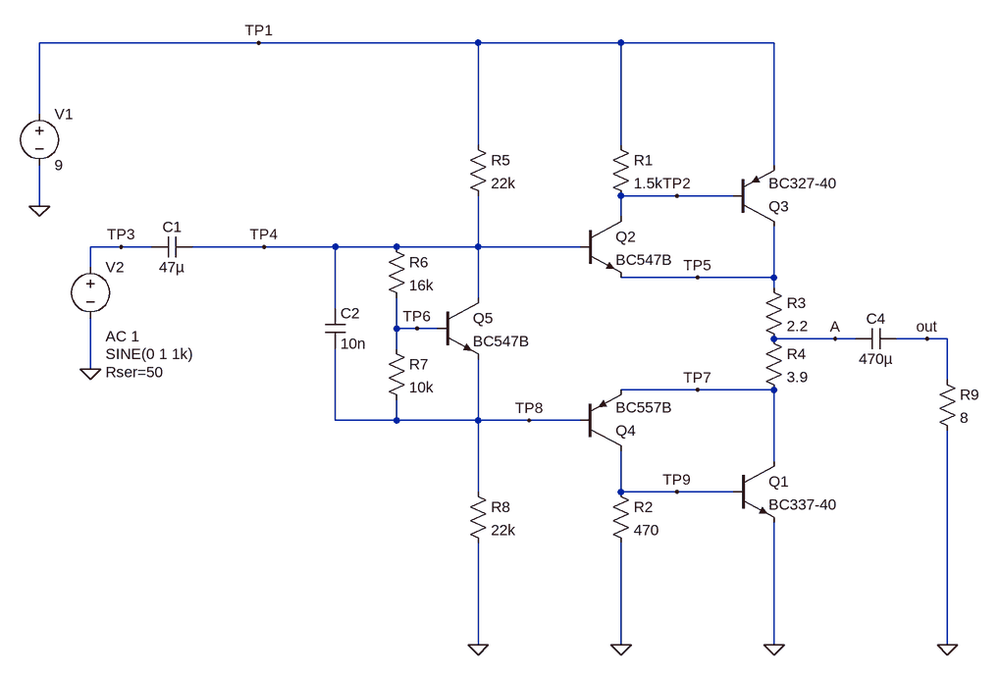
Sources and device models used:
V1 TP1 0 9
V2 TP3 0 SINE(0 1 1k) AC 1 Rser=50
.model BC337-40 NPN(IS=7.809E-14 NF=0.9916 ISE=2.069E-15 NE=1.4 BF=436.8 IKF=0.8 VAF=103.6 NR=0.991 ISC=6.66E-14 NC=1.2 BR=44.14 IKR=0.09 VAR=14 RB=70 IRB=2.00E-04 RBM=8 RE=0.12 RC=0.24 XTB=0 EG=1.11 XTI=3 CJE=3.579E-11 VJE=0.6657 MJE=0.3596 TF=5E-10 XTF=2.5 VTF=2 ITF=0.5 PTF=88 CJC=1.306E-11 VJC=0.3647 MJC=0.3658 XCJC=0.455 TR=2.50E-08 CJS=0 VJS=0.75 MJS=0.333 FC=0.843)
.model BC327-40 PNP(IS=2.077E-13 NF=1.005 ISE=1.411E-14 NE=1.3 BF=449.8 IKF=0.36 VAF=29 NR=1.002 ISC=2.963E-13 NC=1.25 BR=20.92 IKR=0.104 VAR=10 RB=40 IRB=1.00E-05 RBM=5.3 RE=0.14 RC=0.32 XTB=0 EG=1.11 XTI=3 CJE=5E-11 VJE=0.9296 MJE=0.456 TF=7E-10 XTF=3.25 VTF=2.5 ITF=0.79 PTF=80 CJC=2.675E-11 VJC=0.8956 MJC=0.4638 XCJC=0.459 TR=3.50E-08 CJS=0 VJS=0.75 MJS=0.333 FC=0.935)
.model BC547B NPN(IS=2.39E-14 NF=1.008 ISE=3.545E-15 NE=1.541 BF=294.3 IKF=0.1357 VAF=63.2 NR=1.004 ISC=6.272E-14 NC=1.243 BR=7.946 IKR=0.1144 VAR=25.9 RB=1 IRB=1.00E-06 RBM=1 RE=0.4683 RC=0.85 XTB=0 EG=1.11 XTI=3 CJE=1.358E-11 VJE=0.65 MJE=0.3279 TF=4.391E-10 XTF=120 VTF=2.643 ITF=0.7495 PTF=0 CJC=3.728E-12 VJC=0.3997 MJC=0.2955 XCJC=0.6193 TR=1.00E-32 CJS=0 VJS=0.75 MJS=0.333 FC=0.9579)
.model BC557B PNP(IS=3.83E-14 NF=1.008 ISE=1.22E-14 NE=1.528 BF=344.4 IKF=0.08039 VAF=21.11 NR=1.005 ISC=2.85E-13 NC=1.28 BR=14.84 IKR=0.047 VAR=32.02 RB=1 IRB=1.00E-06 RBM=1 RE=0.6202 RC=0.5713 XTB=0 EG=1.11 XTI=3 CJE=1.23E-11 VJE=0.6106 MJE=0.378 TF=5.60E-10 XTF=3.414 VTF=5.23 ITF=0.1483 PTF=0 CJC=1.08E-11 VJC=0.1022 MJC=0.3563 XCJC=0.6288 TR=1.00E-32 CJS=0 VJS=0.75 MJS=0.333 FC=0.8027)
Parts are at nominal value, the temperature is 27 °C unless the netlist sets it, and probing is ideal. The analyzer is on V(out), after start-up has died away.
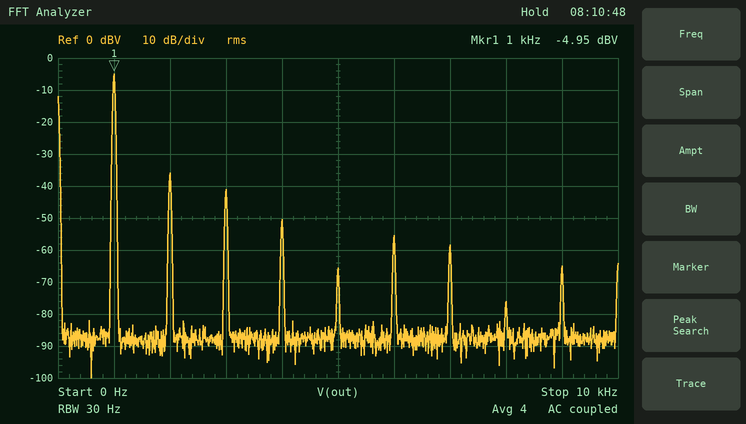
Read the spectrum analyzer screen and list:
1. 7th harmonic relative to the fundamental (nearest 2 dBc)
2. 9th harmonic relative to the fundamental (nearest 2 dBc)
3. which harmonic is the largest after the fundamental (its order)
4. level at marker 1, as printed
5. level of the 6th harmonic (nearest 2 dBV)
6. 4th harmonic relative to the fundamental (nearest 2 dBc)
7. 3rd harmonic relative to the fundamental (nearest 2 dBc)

-54 dBc
-60 dBc
2
-4.95 dBV
-56 dBV
-46 dBc
-36 dBc
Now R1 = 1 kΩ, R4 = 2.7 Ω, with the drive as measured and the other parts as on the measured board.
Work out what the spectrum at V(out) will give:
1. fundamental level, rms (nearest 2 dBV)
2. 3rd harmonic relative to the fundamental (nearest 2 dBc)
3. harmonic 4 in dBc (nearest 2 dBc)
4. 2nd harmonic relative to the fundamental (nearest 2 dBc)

-4 dBV
-44 dBc
-48 dBc
-40 dBc
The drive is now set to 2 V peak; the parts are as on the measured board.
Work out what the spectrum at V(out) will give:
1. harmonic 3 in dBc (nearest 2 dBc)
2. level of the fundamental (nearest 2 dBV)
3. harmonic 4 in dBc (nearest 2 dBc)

-34 dBc
0 dBV
-42 dBc
